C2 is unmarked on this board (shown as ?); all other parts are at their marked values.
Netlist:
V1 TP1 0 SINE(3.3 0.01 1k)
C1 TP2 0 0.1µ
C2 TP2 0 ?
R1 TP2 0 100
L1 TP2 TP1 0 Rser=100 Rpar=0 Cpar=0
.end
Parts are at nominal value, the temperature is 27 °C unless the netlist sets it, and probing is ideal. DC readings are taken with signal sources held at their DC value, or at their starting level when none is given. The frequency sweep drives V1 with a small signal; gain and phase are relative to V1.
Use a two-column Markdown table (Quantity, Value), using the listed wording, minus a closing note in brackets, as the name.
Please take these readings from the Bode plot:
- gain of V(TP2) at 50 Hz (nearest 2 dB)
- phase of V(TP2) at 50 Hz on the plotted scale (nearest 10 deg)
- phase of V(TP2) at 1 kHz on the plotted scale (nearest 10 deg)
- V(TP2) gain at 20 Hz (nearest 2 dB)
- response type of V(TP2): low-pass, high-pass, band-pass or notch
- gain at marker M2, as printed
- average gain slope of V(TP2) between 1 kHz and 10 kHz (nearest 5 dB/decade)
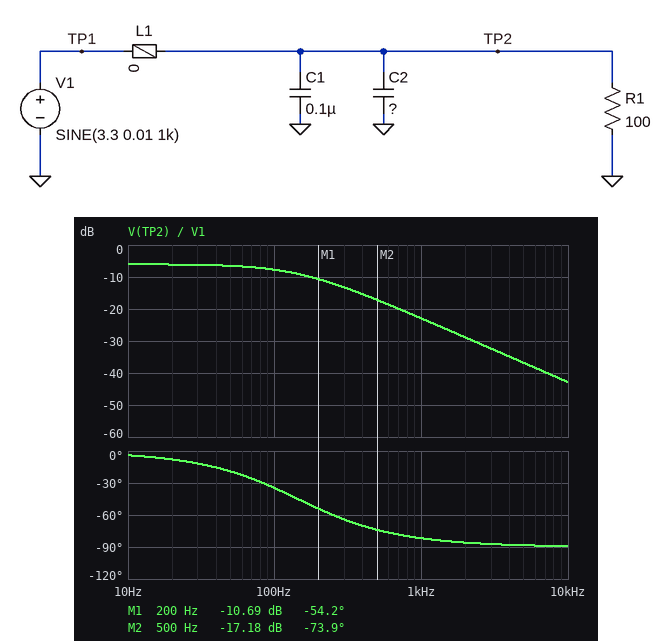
| Quantity | Value |
|---|---|
| gain of V(TP2) at 50 Hz | -6 dB |
| phase of V(TP2) at 50 Hz on the plotted scale | -20 deg |
| phase of V(TP2) at 1 kHz on the plotted scale | -80 deg |
| V(TP2) gain at 20 Hz | -6 dB |
| response type of V(TP2): low-pass, high-pass, band-pass or notch | low-pass |
| gain at marker M2, as printed | -17.18 dB |
| average gain slope of V(TP2) between 1 kHz and 10 kHz | -20 dB/decade |
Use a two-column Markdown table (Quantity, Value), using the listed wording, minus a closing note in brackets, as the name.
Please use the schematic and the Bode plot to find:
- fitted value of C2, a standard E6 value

| Quantity | Value |
|---|---|
| fitted value of C2, a standard E6 value | 22 µF |
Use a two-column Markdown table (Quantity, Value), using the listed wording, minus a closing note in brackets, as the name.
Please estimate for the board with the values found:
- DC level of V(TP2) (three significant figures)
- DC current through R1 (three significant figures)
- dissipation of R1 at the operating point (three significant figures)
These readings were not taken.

| Quantity | Value |
|---|---|
| DC level of V(TP2) | 1.65 V |
| DC current through R1 | 16.5 mA |
| dissipation of R1 at the operating point | 27.2 mW |
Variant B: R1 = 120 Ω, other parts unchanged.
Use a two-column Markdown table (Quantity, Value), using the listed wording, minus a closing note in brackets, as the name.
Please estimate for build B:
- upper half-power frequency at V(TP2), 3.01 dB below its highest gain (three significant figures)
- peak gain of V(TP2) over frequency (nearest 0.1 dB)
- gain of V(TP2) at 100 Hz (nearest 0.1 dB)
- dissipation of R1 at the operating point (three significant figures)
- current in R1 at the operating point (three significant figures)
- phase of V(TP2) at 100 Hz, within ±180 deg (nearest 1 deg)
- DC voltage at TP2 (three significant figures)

| Quantity | Value |
|---|---|
| upper half-power frequency at V(TP2), 3.01 dB below its highest gain | 132 Hz |
| peak gain of V(TP2) over frequency | -5.3 dB |
| gain of V(TP2) at 100 Hz | -7.2 dB |
| dissipation of R1 at the operating point | 27.0 mW |
| current in R1 at the operating point | 15.0 mA |
| phase of V(TP2) at 100 Hz, within ±180 deg | -37 deg |
| DC voltage at TP2 | 1.80 V |
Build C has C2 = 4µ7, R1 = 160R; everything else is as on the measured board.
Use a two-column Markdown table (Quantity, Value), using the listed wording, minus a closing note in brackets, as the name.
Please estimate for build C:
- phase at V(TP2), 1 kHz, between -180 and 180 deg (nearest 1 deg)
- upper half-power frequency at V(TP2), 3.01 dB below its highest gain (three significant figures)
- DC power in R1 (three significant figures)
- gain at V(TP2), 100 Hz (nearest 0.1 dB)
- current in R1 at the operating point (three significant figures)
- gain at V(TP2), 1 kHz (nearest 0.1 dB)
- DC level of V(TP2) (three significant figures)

| Quantity | Value |
|---|---|
| phase at V(TP2), 1 kHz, between -180 and 180 deg | -62 deg |
| upper half-power frequency at V(TP2), 3.01 dB below its highest gain | 539 Hz |
| DC power in R1 | 25.8 mW |
| gain at V(TP2), 100 Hz | -4.4 dB |
| current in R1 at the operating point | 12.7 mA |
| gain at V(TP2), 1 kHz | -10.7 dB |
| DC level of V(TP2) | 2.03 V |
